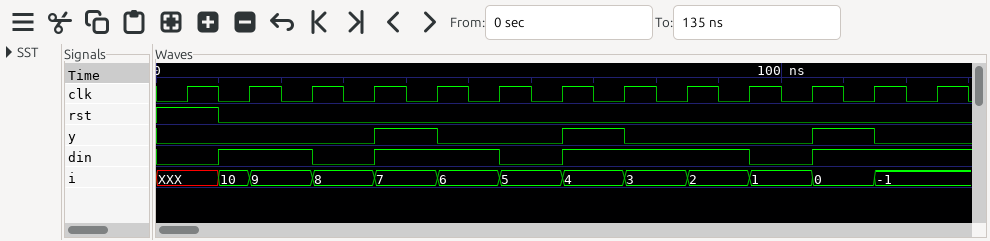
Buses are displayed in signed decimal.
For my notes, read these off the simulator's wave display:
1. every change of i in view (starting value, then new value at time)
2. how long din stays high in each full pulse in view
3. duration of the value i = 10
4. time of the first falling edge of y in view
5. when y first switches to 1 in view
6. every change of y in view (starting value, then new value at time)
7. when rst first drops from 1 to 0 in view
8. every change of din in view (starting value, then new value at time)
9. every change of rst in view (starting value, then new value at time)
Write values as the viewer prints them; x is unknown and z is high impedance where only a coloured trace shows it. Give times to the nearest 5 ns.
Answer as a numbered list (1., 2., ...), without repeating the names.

1. XXX, 10 at 10 ns, 9 at 15 ns, 8 at 25 ns, 7 at 35 ns, 6 at 45 ns, 5 at 55 ns, 4 at 65 ns, 3 at 75 ns, 2 at 85 ns, 1 at 95 ns, 0 at 105 ns, -1 at 115 ns
2. 15 ns, 20 ns, 30 ns
3. 5 ns
4. 45 ns
5. 35 ns
6. 0, 1 at 35 ns, 0 at 45 ns, 1 at 65 ns, 0 at 75 ns, 1 at 105 ns, 0 at 115 ns
7. 10 ns
8. 0, 1 at 10 ns, 0 at 25 ns, 1 at 35 ns, 0 at 55 ns, 1 at 65 ns, 0 at 95 ns, 1 at 105 ns
9. 1, 0 at 10 ns
